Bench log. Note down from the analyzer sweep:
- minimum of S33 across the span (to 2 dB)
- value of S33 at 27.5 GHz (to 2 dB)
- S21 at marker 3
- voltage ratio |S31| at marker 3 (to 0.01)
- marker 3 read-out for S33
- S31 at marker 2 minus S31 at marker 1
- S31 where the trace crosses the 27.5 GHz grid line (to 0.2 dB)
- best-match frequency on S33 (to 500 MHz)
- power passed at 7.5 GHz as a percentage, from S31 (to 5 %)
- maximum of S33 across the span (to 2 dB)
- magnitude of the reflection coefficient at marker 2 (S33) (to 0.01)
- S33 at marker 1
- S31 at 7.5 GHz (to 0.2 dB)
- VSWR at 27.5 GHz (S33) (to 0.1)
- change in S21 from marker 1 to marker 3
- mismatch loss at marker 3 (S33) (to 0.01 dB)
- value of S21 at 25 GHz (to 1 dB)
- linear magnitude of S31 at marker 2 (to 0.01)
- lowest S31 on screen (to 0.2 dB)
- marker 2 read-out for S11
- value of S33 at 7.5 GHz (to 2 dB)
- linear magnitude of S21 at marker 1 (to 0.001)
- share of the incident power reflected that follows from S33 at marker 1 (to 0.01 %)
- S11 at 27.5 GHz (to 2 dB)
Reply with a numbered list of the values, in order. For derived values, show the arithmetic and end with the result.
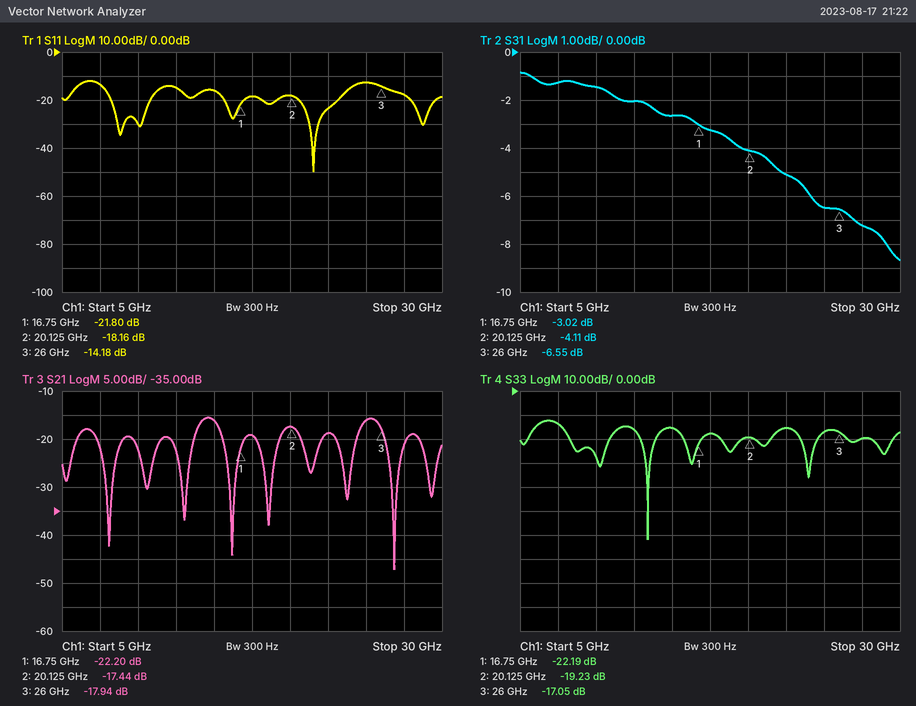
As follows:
1. -62 dB
2. -20 dB
3. -17.94 dB
4. 10^(-6.55/20) ≈ 0.47
5. -17.05 dB
6. -4.11 − (-3.02) = -1.09 dB
7. -7.2 dB
8. 13.5 GHz
9. 10^(-1.2/10) ≈ 75.9 %, so 75 % to the nearest 5 %
10. -12 dB
11. 10^(-19.23/20) ≈ 0.11
12. -22.19 dB
13. -1.2 dB
14. |Γ| = 10^(-20/20) = 0.1000; VSWR = (1 + 0.1000)/(1 − 0.1000) ≈ 1.2
15. -17.94 − (-22.2) = 4.26 dB
16. −10 log10(1 − 10^(-17.05/10)) ≈ 0.09 dB
17. -16 dB
18. 10^(-4.11/20) ≈ 0.62
19. -8.6 dB
20. -18.16 dB
21. -14 dB
22. 10^(-22.2/20) ≈ 0.078
23. 10^(-22.19/10) ≈ 0.60 %
24. -18 dB
